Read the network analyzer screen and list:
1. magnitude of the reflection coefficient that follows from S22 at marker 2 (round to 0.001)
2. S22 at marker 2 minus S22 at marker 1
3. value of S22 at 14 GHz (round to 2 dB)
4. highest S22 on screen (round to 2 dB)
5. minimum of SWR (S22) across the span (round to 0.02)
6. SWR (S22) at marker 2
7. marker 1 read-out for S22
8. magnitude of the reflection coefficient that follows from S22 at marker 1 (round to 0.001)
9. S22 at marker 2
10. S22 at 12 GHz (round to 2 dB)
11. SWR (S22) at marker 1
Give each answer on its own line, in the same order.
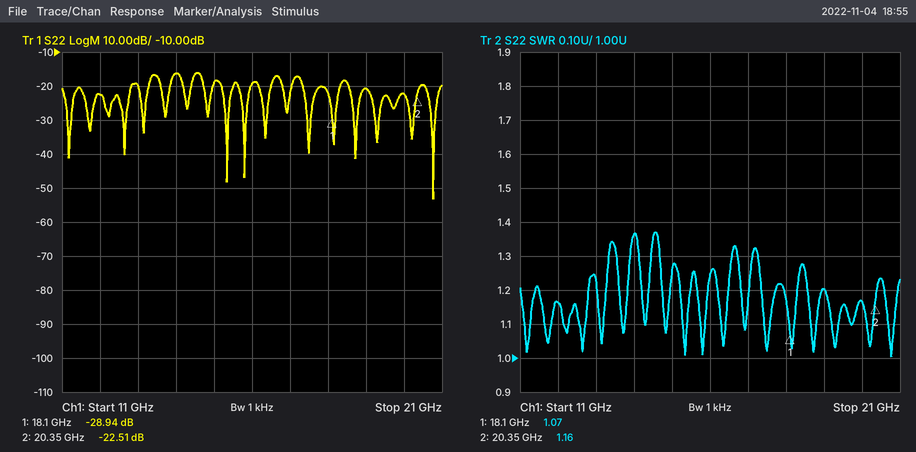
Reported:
0.075
6.43 dB
-16 dB
-16 dB
1.00
1.16
-28.94 dB
0.036
-22.51 dB
-22 dB
1.07
